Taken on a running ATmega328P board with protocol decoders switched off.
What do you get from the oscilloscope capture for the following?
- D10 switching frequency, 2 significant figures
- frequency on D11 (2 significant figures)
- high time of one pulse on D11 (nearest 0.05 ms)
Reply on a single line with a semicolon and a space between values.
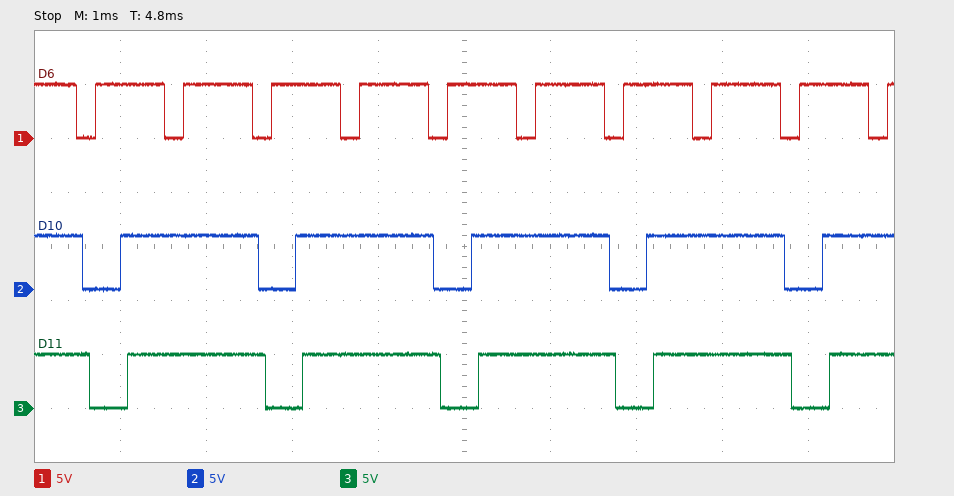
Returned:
490 Hz; 490 Hz; 1.60 ms
